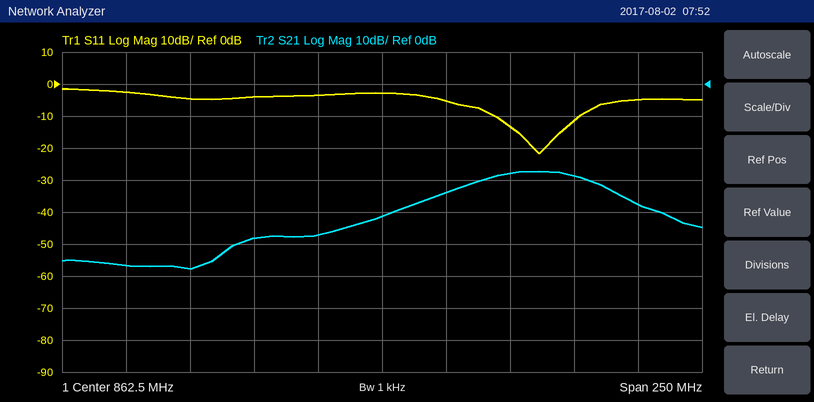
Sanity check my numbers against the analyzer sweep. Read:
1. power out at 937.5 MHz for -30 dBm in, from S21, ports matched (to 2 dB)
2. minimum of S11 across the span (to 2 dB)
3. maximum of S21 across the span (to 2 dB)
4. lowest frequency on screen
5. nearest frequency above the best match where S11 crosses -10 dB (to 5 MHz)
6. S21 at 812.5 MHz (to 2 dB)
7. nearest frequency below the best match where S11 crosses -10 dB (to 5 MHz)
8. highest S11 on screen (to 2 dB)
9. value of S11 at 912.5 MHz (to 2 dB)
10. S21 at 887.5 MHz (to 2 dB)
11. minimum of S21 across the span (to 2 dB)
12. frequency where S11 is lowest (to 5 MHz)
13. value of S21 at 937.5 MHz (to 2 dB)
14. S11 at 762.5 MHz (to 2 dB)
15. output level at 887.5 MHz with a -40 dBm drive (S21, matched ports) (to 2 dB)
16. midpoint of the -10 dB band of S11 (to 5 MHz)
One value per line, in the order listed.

-58 dBm
-22 dB
-28 dB
737.5 MHz
940 MHz
-48 dB
905 MHz
-2 dB
-14 dB
-34 dB
-58 dB
925 MHz
-28 dB
-2 dB
-74 dBm
925 MHz
